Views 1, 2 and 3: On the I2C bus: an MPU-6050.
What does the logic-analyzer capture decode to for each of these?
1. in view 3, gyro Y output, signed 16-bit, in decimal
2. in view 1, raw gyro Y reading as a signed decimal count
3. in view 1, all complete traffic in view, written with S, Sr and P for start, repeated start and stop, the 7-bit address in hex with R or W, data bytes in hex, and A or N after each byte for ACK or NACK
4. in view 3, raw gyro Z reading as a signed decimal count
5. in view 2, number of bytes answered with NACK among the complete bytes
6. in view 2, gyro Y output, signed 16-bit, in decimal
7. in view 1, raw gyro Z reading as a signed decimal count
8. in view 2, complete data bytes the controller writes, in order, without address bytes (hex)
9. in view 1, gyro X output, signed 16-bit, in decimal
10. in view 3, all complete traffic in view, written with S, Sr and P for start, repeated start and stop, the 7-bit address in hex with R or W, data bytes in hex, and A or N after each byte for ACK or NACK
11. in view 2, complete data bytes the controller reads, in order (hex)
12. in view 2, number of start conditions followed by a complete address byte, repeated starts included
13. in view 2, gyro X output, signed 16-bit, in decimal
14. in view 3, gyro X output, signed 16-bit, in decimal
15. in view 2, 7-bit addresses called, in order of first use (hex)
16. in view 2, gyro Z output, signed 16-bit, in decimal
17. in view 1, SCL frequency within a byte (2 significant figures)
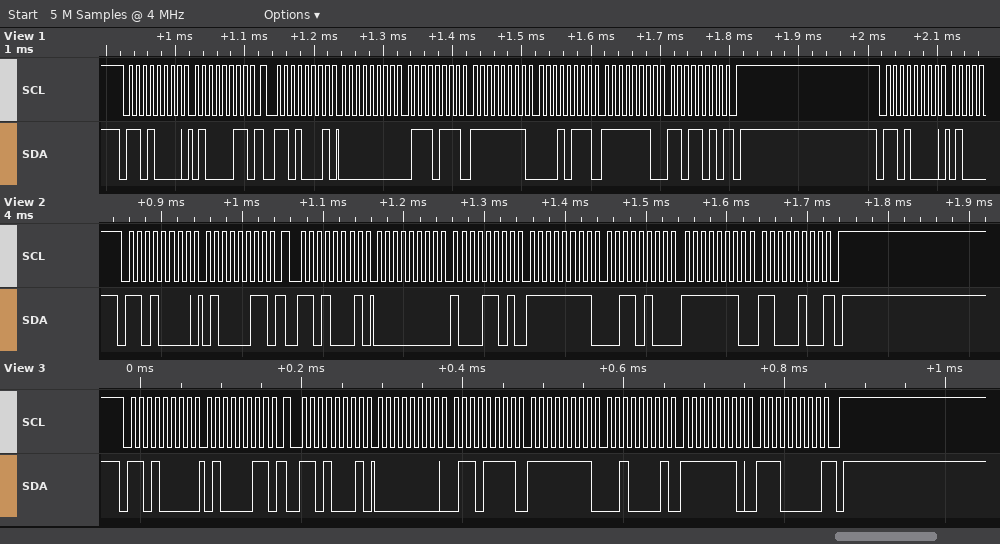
-223
-233
S 68W A 43 A Sr 68R A 00 A 77 A FF A 17 A FE A DA N P S 68W A
-288
1
-204
-294
43
119
S 68W A 43 A Sr 68R A 00 A 6F A FF A 21 A FE A E0 N P
00 8D FF 34 FE C4
2
141
111
0x68
-316
100 kHz
